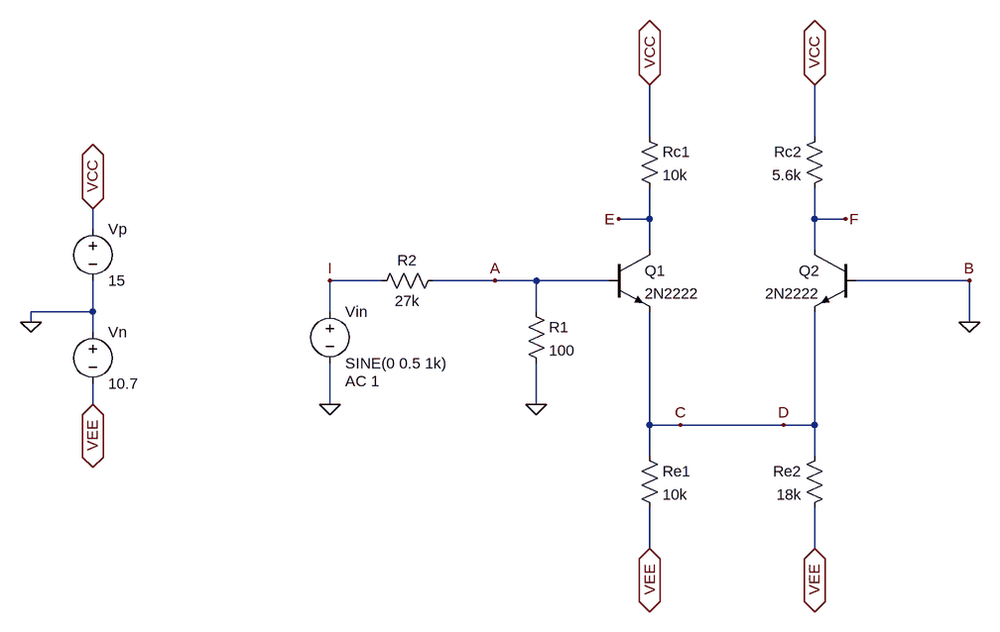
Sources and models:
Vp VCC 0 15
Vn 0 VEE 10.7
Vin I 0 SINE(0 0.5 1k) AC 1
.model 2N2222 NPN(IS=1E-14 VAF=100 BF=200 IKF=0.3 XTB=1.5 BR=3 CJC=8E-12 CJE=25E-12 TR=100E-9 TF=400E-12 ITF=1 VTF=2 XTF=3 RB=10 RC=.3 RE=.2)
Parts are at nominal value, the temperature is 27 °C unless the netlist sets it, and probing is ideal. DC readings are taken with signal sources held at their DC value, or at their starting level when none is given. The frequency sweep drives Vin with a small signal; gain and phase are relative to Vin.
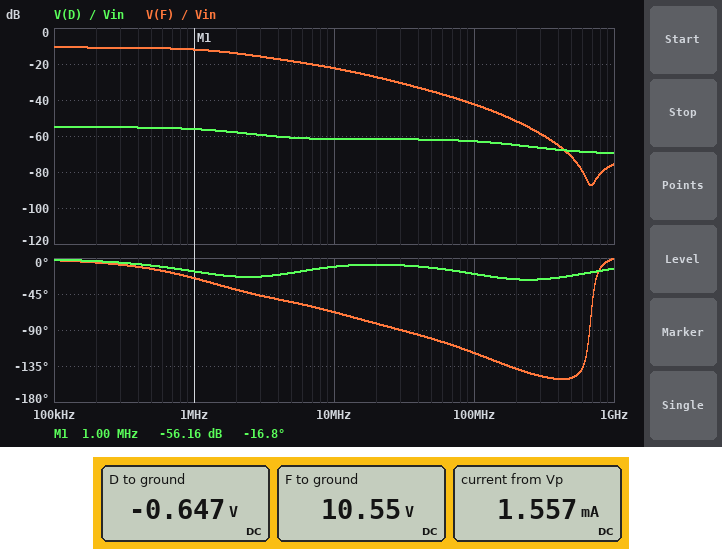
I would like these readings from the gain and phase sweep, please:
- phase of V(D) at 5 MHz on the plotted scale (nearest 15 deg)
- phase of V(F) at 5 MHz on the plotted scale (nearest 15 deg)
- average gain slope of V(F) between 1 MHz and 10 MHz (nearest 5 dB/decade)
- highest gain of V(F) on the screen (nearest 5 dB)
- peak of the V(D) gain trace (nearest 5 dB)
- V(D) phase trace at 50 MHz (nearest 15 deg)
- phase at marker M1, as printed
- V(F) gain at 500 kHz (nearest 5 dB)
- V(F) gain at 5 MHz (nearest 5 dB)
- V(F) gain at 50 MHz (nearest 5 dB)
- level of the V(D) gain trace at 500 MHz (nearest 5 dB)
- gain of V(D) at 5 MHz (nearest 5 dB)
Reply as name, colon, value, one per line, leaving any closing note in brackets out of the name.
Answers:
phase of V(D) at 5 MHz on the plotted scale: -15 deg
phase of V(F) at 5 MHz on the plotted scale: -60 deg
average gain slope of V(F) between 1 MHz and 10 MHz: -10 dB/decade
highest gain of V(F) on the screen: -10 dB
peak of the V(D) gain trace: -55 dB
V(D) phase trace at 50 MHz: -15 deg
phase at marker M1, as printed: -16.8 deg
V(F) gain at 500 kHz: -10 dB
V(F) gain at 5 MHz: -20 dB
V(F) gain at 50 MHz: -35 dB
level of the V(D) gain trace at 500 MHz: -70 dB
gain of V(D) at 5 MHz: -60 dB
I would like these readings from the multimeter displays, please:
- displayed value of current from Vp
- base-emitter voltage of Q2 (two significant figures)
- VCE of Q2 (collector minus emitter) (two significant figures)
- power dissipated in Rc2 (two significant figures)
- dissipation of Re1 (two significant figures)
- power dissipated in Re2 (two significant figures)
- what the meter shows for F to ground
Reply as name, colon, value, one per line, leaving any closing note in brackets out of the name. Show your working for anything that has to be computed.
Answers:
displayed value of current from Vp: 1.557 mA
base-emitter voltage of Q2: 0 V - (-647 mV) = 650 mV
VCE of Q2 (collector minus emitter): 10.55 V - (-647 mV) = 11 V
power dissipated in Rc2: (15 V - 10.55 V)^2 / 5.6 kΩ = 3.5 mW
dissipation of Re1: (-647 mV - (-10.7 V))^2 / 10 kΩ = 10 mW
power dissipated in Re2: (-647 mV - (-10.7 V))^2 / 18 kΩ = 5.6 mW
what the meter shows for F to ground: 10.55 V
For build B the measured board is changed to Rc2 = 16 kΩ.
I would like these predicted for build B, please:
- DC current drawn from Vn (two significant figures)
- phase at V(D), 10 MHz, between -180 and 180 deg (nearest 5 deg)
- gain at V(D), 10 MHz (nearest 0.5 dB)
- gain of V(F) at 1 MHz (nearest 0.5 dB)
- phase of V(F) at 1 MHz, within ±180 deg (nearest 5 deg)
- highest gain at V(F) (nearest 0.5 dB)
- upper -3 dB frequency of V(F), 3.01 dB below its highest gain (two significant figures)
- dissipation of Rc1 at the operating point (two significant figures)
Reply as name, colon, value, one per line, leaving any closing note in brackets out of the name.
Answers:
DC current drawn from Vn: 1.6 mA
phase at V(D), 10 MHz, between -180 and 180 deg: -15 deg
gain at V(D), 10 MHz: -61.0 dB
gain of V(F) at 1 MHz: -4.0 dB
phase of V(F) at 1 MHz, within ±180 deg: -45 deg
highest gain at V(F): -2.0 dB
upper -3 dB frequency of V(F), 3.01 dB below its highest gain: 1.2 MHz
dissipation of Rc1 at the operating point: 6.2 mW
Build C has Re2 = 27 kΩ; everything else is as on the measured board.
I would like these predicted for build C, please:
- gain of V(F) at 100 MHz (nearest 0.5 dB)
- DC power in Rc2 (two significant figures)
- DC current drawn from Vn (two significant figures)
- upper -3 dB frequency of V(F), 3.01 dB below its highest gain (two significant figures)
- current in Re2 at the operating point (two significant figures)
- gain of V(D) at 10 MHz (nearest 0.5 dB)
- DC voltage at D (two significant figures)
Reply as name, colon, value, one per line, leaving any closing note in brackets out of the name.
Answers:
gain of V(F) at 100 MHz: -43.0 dB
DC power in Rc2: 2.7 mW
DC current drawn from Vn: 1.4 mA
upper -3 dB frequency of V(F), 3.01 dB below its highest gain: 2.1 MHz
current in Re2 at the operating point: 370 µA
gain of V(D) at 10 MHz: -61.0 dB
DC voltage at D: -640 mV
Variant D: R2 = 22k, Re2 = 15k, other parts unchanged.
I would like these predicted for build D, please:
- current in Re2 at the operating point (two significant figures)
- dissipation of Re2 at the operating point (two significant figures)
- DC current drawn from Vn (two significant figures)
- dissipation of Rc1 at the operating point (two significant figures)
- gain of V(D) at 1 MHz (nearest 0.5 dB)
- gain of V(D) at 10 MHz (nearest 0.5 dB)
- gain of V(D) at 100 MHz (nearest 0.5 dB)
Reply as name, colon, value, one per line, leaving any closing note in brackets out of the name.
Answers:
current in Re2 at the operating point: 670 µA
dissipation of Re2 at the operating point: 6.7 mW
DC current drawn from Vn: 1.7 mA
dissipation of Rc1 at the operating point: 6.6 mW
gain of V(D) at 1 MHz: -54.5 dB
gain of V(D) at 10 MHz: -60.0 dB
gain of V(D) at 100 MHz: -61.5 dB
